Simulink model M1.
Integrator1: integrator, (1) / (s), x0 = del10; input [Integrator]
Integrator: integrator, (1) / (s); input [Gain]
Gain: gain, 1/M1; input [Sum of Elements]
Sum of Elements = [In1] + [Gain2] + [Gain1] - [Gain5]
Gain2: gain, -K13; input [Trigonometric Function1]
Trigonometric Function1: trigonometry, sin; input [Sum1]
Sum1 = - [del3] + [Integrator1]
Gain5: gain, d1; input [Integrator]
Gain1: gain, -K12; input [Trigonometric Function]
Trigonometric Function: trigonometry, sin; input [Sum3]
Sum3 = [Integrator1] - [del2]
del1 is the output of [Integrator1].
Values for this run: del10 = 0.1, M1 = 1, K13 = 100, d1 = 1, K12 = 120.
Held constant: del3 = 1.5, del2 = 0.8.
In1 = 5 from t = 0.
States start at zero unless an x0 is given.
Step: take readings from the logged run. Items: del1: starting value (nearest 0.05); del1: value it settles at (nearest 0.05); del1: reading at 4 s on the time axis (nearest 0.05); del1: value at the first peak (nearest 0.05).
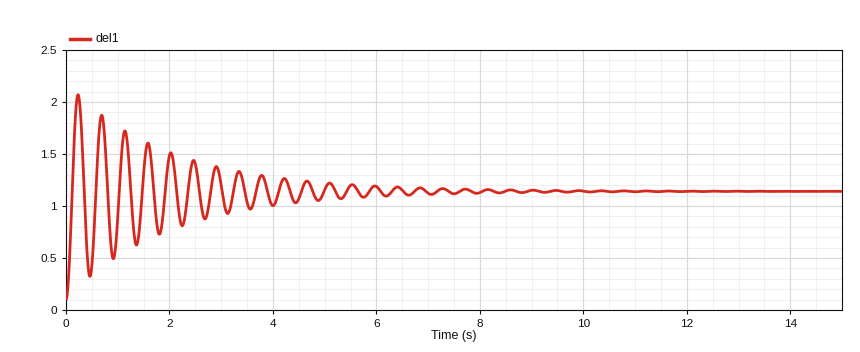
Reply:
0.10
1.15
1.00
2.05
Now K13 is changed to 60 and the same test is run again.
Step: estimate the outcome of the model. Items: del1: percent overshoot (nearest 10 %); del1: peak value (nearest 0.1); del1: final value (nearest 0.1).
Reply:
90 %
1.9
1.1
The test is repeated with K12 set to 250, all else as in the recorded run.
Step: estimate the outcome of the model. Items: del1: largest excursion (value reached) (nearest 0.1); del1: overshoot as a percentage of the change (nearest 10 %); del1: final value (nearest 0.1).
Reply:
1.8
90 %
1.0
